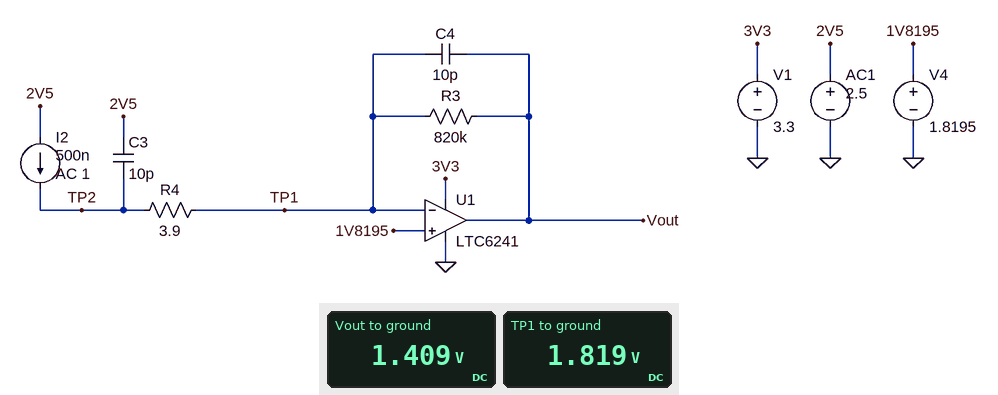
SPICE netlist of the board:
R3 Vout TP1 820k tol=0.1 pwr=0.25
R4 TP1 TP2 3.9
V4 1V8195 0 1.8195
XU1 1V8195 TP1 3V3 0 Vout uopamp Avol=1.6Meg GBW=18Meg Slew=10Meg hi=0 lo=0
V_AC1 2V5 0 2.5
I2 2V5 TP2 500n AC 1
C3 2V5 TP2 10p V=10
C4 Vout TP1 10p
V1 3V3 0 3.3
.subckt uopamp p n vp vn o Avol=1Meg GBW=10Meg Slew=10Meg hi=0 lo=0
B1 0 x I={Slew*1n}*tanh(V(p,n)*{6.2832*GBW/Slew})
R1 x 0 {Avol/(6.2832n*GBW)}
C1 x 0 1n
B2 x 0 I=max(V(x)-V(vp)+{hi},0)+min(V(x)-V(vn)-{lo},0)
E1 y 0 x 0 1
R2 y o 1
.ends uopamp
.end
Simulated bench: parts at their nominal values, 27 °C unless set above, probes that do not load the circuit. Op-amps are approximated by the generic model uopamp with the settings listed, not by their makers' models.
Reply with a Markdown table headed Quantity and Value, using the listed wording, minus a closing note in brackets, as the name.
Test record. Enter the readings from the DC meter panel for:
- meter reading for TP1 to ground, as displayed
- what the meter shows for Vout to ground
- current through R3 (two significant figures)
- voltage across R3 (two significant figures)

| Quantity | Value |
|---|---|
| meter reading for TP1 to ground, as displayed | 1.819 V |
| what the meter shows for Vout to ground | 1.409 V |
| current through R3 | 500 nA |
| voltage across R3 | 410 mV |
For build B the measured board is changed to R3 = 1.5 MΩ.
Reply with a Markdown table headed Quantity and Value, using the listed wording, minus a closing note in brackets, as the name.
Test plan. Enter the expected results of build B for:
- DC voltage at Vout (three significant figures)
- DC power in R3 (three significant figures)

| Quantity | Value |
|---|---|
| DC voltage at Vout | 1.07 V |
| DC power in R3 | 375 nW |
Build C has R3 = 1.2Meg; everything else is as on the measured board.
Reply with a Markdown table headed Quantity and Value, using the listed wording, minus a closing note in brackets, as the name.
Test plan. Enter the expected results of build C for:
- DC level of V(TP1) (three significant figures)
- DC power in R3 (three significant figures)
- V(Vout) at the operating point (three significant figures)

| Quantity | Value |
|---|---|
| DC level of V(TP1) | 1.82 V |
| DC power in R3 | 300 nW |
| V(Vout) at the operating point | 1.22 V |
